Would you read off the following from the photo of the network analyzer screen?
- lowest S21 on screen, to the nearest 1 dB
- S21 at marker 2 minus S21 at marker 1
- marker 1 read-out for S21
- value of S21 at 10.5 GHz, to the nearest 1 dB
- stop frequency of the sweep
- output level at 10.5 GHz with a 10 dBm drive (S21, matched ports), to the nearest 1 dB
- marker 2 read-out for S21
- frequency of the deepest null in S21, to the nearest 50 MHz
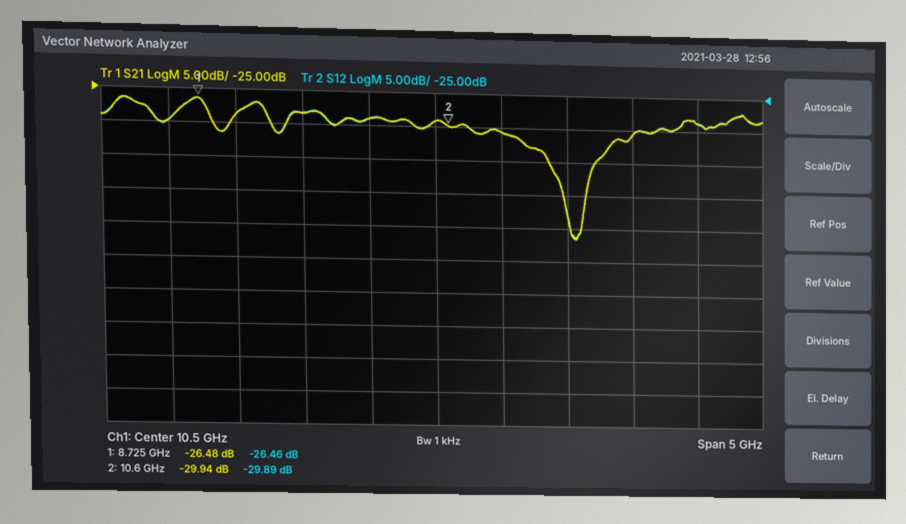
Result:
-47 dB
-3.46 dB
-26.48 dB
-29 dB
13 GHz
-19 dBm
-29.94 dB
11.55 GHz
